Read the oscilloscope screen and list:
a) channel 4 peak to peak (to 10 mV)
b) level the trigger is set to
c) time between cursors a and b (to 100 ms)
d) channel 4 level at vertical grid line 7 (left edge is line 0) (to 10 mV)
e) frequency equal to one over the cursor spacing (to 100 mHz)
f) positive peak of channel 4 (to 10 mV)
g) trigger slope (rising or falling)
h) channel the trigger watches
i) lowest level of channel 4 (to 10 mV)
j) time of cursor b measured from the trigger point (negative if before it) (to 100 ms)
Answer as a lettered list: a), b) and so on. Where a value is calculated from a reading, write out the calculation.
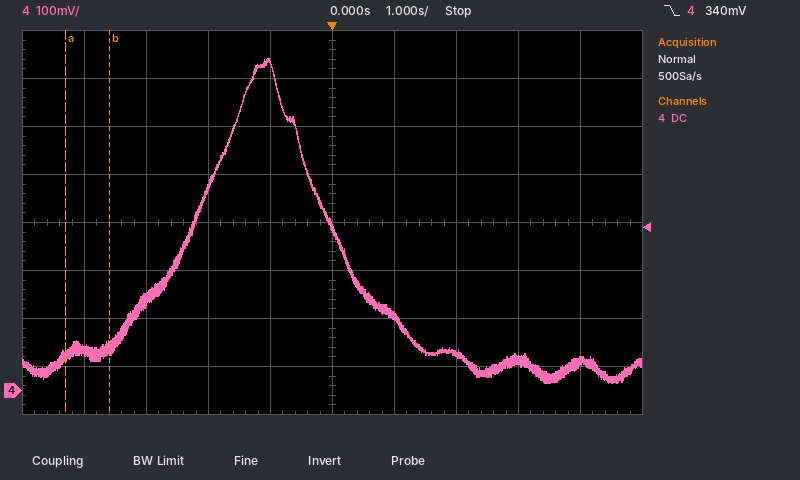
a) 690 mV − (10 mV) = 680 mV
b) 340 mV
c) 700 ms
d) 80 mV
e) 1 / 700 ms ≈ 1.4 Hz
f) 690 mV
g) falling
h) channel 4
i) 10 mV
j) -3.6 s
